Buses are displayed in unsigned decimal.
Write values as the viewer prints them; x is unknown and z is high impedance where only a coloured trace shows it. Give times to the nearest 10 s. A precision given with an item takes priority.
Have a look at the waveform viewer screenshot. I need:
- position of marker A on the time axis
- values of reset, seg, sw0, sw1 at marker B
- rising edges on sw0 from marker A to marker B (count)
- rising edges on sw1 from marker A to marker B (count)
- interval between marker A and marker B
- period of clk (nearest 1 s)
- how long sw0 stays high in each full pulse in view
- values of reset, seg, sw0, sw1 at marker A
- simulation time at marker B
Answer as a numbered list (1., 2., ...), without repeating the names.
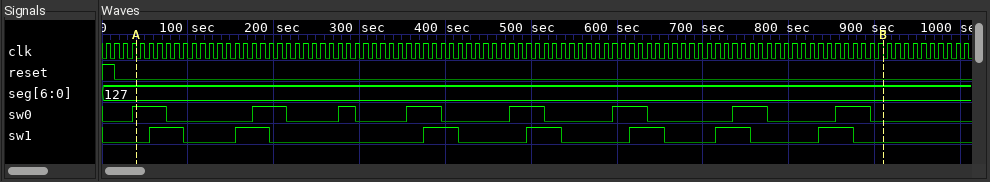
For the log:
1. 40 s
2. reset=0, seg=127, sw0=0, sw1=0
3. 7
4. 7
5. 870 s
6. 10 s
7. 40 s, 40 s, 20 s, 40 s, 40 s, 40 s, 40 s, 40 s
8. reset=0, seg=127, sw0=1, sw1=0
9. 910 s
